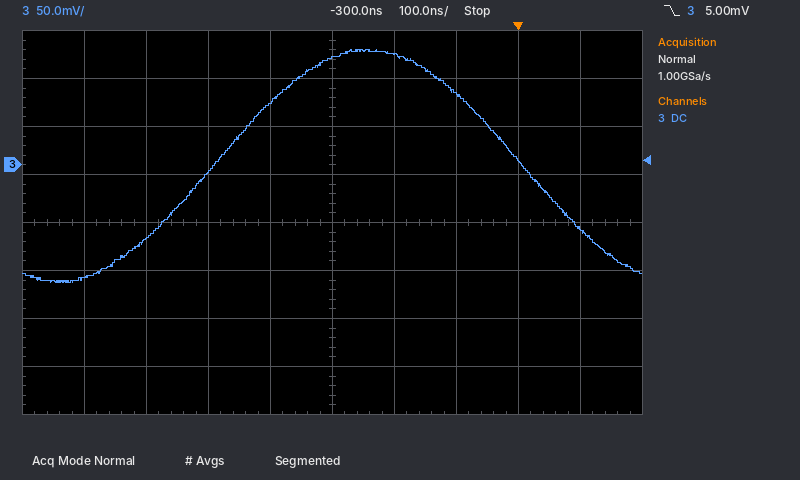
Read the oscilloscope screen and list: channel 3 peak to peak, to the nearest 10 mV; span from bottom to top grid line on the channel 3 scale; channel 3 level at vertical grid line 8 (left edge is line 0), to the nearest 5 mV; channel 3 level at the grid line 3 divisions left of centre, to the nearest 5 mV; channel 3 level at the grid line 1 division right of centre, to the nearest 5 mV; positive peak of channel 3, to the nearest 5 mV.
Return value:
240 mV
400 mV
5 mV
-75 mV
115 mV
120 mV
